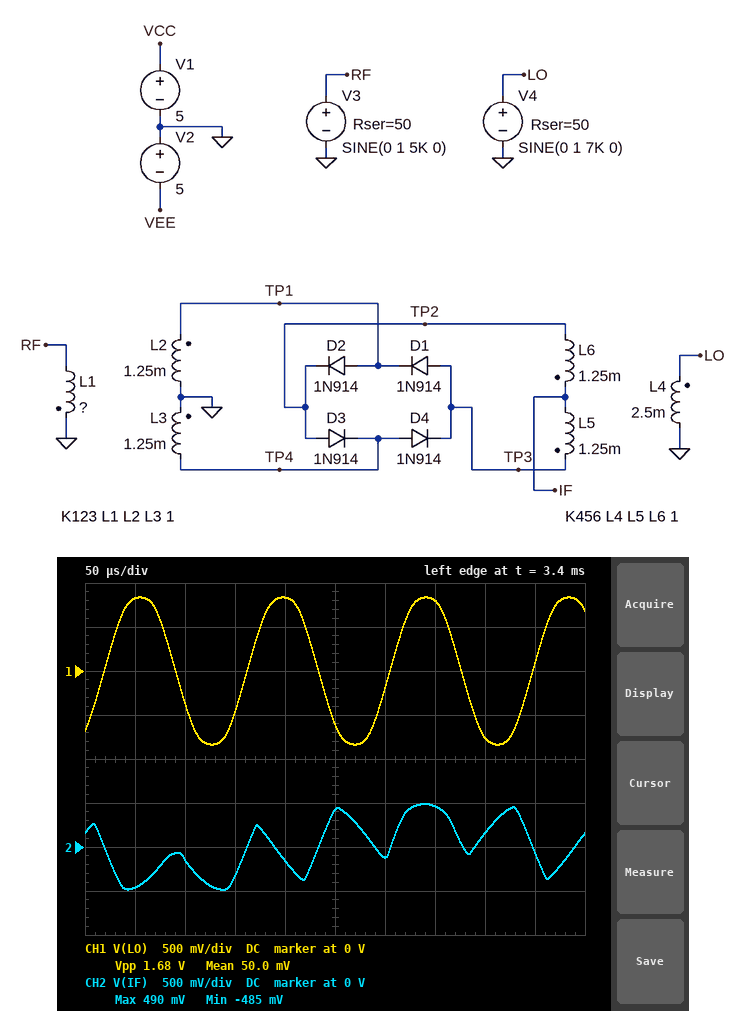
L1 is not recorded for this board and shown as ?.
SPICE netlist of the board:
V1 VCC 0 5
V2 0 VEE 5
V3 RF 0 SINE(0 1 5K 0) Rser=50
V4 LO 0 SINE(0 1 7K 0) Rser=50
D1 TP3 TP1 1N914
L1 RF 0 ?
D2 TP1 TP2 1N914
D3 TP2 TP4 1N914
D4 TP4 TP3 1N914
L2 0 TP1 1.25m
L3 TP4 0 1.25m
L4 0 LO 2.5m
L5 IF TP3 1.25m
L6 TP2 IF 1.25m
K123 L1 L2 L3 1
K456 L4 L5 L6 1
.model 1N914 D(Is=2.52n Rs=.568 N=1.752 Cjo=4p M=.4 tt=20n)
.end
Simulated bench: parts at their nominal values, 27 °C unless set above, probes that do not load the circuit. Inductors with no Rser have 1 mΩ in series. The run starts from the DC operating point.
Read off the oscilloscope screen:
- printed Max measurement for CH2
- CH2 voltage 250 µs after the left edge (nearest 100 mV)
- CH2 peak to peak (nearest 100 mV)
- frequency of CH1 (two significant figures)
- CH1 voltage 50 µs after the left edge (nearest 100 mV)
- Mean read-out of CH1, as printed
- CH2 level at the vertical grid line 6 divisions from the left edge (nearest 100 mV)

490 mV
400 mV
1.0 V
7.0 kHz
800 mV
50.0 mV
-100 mV
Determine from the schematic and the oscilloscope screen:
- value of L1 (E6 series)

4.7 mH
